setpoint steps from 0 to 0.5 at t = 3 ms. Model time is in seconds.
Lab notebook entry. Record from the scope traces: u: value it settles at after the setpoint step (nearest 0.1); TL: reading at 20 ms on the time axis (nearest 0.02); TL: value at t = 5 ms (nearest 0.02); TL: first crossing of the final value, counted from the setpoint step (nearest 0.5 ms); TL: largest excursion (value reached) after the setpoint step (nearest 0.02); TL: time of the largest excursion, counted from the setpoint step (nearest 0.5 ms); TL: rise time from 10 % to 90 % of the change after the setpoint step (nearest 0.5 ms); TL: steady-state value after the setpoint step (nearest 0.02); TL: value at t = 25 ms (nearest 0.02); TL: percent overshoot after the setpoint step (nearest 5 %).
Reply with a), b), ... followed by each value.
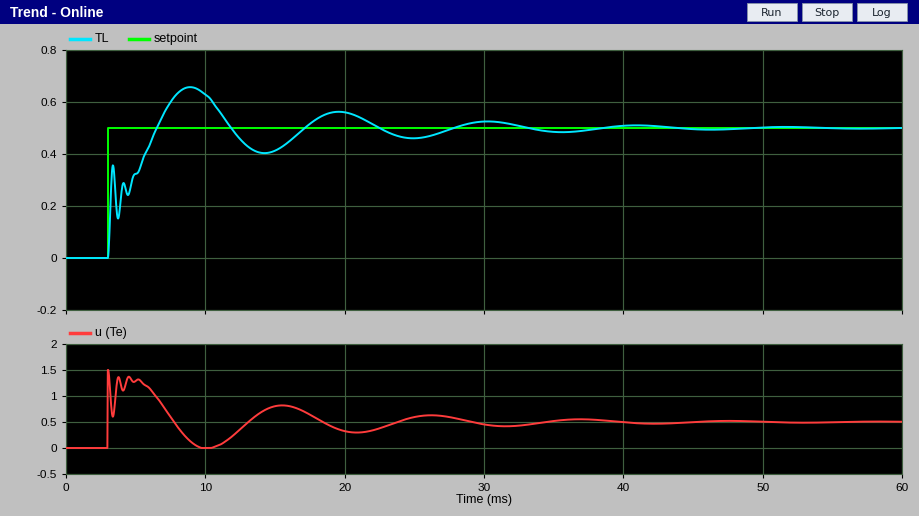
a) 0.5
b) 0.56
c) 0.32
d) 3.5 ms
e) 0.66
f) 6.0 ms
g) 3.0 ms
h) 0.50
i) 0.46
j) 30 %
